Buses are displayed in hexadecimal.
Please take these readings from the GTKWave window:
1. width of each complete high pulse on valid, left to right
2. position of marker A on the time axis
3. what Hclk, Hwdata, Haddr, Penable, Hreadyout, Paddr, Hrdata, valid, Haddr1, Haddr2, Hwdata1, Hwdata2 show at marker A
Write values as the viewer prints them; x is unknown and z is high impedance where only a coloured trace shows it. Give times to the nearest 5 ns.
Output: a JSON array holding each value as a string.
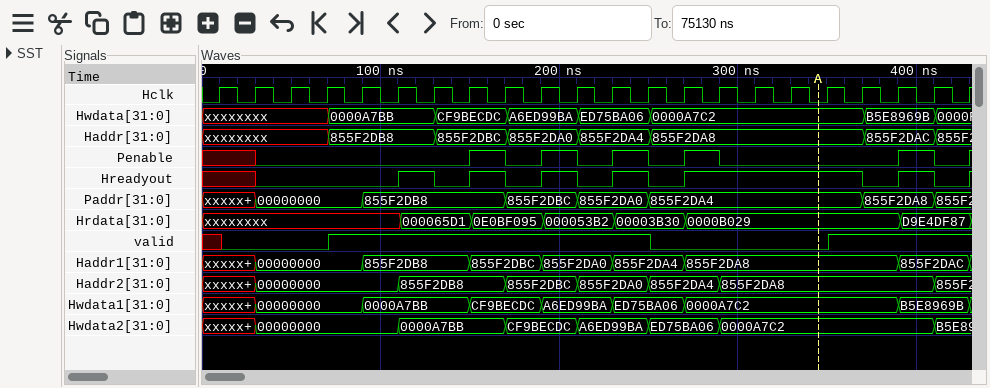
["180 ns", "345 ns", "Hclk=0, Hwdata=0000A7C2, Haddr=855F2DA8, Penable=0, Hreadyout=1, Paddr=855F2DA4, Hrdata=0000B029, valid=0, Haddr1=855F2DA8, Haddr2=855F2DA8, Hwdata1=0000A7C2, Hwdata2=0000A7C2"]
